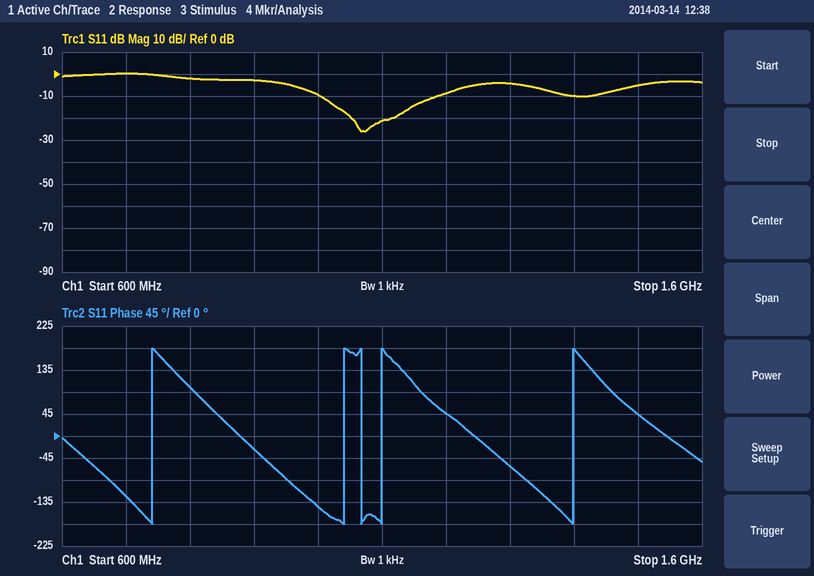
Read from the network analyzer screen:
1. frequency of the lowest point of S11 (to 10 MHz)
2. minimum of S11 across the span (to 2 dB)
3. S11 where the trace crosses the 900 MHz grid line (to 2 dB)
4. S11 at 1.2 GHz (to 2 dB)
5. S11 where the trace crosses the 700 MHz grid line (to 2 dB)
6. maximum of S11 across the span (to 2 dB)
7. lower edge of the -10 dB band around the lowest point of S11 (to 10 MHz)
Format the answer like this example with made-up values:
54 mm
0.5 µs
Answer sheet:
1.07 GHz
-26 dB
-2 dB
-8 dB
0 dB
0 dB
1.00 GHz
